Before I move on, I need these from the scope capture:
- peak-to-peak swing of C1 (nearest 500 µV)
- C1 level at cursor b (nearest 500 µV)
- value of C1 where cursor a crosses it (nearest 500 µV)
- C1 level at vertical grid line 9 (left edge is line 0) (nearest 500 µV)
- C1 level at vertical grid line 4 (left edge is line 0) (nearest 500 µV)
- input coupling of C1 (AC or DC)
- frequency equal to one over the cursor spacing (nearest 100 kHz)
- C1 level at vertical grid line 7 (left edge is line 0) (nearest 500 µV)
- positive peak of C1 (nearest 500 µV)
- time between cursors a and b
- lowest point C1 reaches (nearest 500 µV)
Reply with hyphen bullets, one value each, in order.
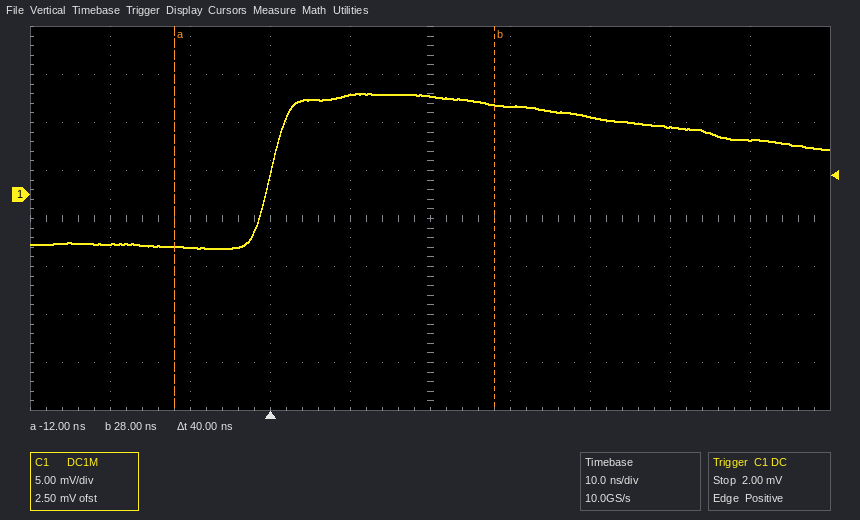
- 16.0 mV
- 9.5 mV
- -5.5 mV
- 5.5 mV
- 10.5 mV
- DC
- 25.0 MHz
- 8.0 mV
- 10.5 mV
- 40 ns
- -5.5 mV
